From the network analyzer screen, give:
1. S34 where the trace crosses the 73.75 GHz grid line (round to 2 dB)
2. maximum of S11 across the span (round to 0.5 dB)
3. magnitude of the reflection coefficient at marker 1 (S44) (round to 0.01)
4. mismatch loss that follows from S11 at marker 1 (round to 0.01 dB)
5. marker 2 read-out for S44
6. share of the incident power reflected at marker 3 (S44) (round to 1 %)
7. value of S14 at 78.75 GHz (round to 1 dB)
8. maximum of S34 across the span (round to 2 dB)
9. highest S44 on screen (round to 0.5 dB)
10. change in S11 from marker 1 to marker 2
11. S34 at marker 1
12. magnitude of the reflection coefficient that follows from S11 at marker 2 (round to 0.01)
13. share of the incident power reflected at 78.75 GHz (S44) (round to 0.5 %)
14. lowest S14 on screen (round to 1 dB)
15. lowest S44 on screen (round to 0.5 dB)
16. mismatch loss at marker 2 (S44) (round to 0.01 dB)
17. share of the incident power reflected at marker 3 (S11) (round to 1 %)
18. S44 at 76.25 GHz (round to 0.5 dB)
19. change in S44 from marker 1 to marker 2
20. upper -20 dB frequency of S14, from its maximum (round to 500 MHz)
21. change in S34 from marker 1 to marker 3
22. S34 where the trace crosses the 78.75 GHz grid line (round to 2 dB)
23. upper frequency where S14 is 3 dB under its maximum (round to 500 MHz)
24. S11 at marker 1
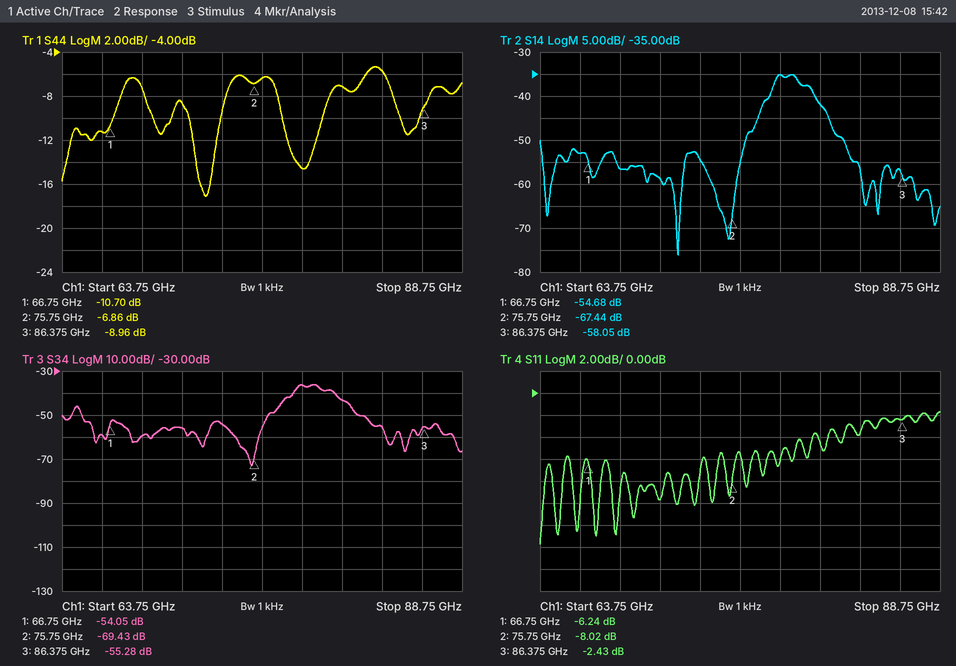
-54 dB
-1.5 dB
0.29
1.18 dB
-6.86 dB
13 %
-35 dB
-36 dB
-5.5 dB
-1.78 dB
-54.05 dB
0.40
3.5 %
-76 dB
-17.0 dB
1.00 dB
57 %
-6.5 dB
3.84 dB
83.5 GHz
-1.23 dB
-36 dB
80.5 GHz
-6.24 dB
